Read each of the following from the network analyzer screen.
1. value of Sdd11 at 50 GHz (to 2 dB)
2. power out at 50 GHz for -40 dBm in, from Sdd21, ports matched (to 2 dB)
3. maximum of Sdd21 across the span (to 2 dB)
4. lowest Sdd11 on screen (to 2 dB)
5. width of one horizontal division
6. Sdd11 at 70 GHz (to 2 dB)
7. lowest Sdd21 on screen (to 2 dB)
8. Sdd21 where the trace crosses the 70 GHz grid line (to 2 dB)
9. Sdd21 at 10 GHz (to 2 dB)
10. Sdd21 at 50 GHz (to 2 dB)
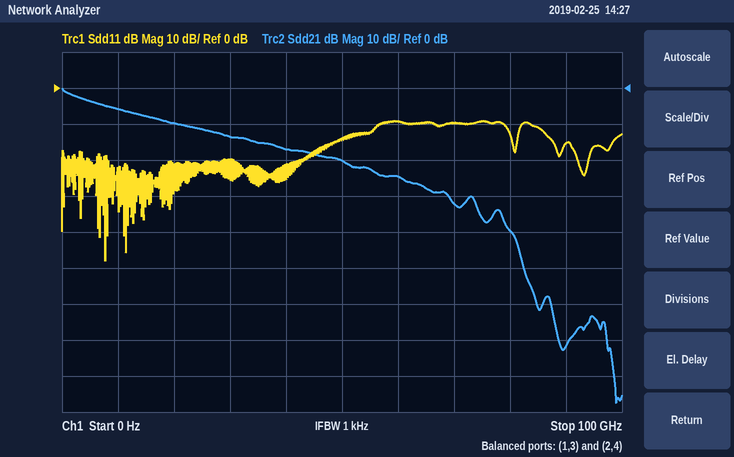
-14 dB
-60 dBm
0 dB
-48 dB
10 GHz
-10 dB
-88 dB
-32 dB
-6 dB
-20 dB
